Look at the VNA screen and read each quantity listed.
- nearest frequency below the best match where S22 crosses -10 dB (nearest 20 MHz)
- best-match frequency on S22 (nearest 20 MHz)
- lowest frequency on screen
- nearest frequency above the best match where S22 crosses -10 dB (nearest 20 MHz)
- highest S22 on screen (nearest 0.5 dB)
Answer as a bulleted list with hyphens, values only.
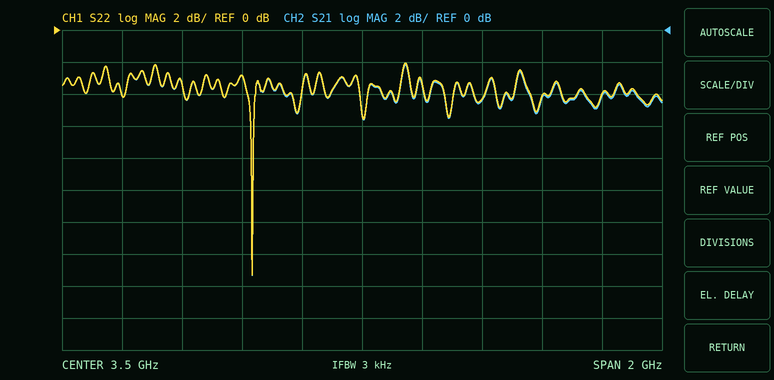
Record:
- 3.14 GHz
- 3.14 GHz
- 2.5 GHz
- 3.14 GHz
- -2.0 dB
